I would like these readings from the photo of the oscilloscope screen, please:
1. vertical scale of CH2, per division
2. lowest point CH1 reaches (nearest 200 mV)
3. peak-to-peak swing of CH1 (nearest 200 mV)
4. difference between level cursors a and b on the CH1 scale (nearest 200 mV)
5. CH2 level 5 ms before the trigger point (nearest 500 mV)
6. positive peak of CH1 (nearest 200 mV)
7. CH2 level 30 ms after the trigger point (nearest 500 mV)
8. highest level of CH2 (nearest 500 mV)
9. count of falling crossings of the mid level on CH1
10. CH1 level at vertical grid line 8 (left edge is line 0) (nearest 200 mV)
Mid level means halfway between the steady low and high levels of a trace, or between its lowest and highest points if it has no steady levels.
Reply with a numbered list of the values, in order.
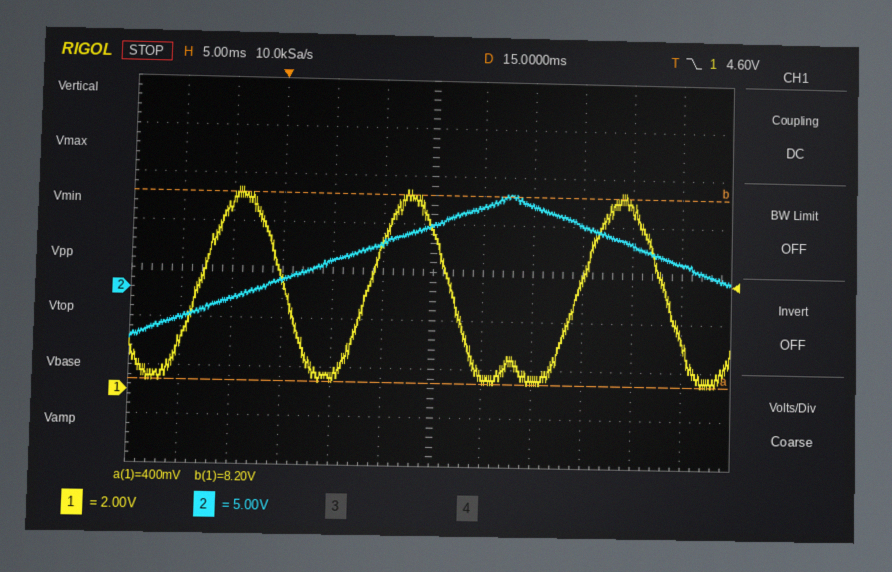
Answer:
1. 5 V
2. 400 mV
3. 8.0 V
4. 7.8 V
5. -1.0 V
6. 8.4 V
7. 7.0 V
8. 10.0 V
9. 3
10. 600 mV
